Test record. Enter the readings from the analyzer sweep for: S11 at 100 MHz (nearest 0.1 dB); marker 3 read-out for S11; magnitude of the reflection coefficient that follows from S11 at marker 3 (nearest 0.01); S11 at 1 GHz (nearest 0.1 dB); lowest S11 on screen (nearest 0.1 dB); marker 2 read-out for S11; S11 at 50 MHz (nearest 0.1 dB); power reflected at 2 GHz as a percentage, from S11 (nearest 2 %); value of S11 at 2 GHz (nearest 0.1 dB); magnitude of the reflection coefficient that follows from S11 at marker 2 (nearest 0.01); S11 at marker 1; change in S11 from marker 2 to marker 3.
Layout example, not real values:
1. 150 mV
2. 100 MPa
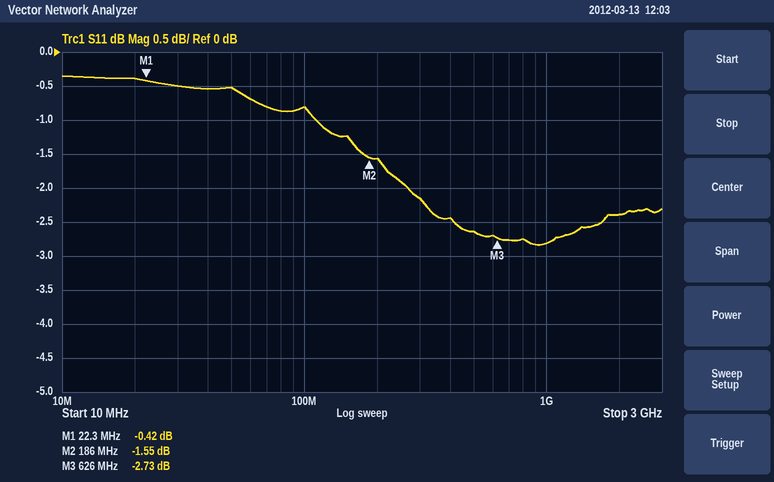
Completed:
1. -0.8 dB
2. -2.73 dB
3. 0.73
4. -2.8 dB
5. -2.8 dB
6. -1.55 dB
7. -0.5 dB
8. 58 %
9. -2.4 dB
10. 0.84
11. -0.42 dB
12. -1.18 dB
